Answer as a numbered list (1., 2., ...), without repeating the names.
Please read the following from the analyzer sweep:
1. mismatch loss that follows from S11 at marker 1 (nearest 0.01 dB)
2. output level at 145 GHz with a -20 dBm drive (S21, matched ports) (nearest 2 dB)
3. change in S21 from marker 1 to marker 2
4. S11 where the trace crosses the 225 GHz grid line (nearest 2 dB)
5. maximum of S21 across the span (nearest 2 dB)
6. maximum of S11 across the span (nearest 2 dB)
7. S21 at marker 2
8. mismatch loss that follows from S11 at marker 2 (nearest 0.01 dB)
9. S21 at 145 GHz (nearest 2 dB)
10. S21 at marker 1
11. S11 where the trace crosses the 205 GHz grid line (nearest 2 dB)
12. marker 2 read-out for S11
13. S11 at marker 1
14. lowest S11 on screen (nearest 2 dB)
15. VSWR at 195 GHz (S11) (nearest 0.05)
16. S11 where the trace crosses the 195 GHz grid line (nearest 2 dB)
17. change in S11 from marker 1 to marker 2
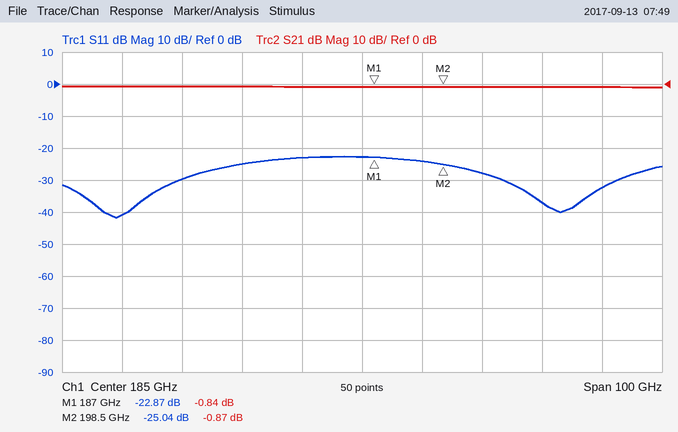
1. 0.02 dB
2. -20 dBm
3. -0.03 dB
4. -32 dB
5. 0 dB
6. -22 dB
7. -0.87 dB
8. 0.01 dB
9. 0 dB
10. -0.84 dB
11. -28 dB
12. -25.04 dB
13. -22.87 dB
14. -42 dB
15. 1.15
16. -24 dB
17. -2.17 dB
